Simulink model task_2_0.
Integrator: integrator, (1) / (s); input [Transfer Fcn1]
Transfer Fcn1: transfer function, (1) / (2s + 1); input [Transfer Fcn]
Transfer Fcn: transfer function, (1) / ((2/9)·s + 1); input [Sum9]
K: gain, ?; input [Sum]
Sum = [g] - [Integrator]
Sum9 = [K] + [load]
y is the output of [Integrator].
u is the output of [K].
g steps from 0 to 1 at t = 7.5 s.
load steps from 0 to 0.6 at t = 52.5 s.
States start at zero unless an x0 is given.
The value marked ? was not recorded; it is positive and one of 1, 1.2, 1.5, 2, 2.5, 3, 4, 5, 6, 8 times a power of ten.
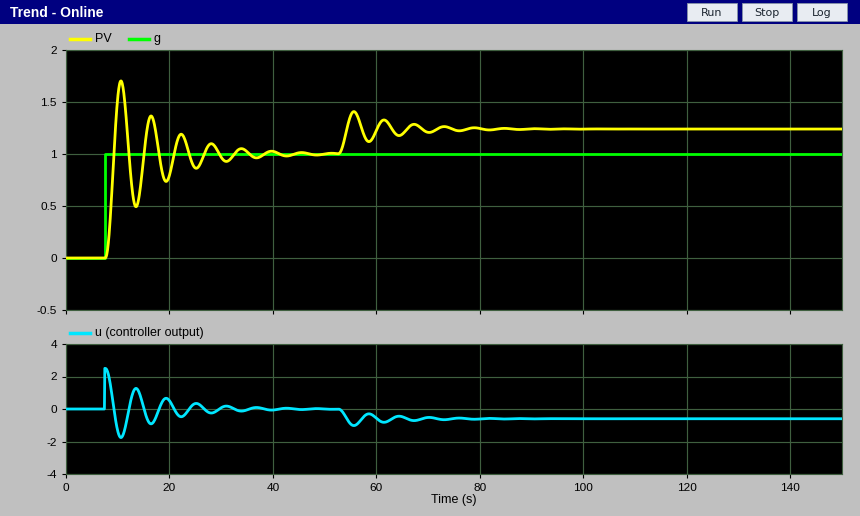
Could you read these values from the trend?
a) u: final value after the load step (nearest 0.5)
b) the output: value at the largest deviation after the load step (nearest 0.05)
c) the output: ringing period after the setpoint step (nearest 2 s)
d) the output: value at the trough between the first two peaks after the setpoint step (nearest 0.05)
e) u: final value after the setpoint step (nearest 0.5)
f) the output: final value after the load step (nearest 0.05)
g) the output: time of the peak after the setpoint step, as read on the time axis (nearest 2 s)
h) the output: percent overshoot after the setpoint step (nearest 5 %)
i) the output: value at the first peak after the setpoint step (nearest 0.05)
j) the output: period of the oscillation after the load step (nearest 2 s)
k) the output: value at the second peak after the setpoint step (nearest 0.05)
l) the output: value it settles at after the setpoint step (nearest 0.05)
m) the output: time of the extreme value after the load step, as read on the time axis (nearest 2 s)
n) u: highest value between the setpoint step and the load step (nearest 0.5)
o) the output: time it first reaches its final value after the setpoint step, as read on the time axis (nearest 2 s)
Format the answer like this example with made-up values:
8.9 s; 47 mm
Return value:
-0.5; 1.40; 6 s; 0.50; 0.0; 1.25; 10 s; 70 %; 1.70; 6 s; 1.35; 1.00; 56 s; 2.5; 10 s
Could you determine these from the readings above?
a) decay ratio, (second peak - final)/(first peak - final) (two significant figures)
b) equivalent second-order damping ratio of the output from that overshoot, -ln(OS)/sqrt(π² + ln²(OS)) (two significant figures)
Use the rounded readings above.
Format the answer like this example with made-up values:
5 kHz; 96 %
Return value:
0.50; 0.11
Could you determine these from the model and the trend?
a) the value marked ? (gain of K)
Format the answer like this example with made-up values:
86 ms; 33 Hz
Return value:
2.5
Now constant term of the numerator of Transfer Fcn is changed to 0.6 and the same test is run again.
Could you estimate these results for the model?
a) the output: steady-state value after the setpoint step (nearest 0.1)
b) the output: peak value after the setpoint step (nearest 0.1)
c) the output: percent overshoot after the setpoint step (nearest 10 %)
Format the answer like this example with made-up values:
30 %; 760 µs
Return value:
1.0; 1.5; 50 %
